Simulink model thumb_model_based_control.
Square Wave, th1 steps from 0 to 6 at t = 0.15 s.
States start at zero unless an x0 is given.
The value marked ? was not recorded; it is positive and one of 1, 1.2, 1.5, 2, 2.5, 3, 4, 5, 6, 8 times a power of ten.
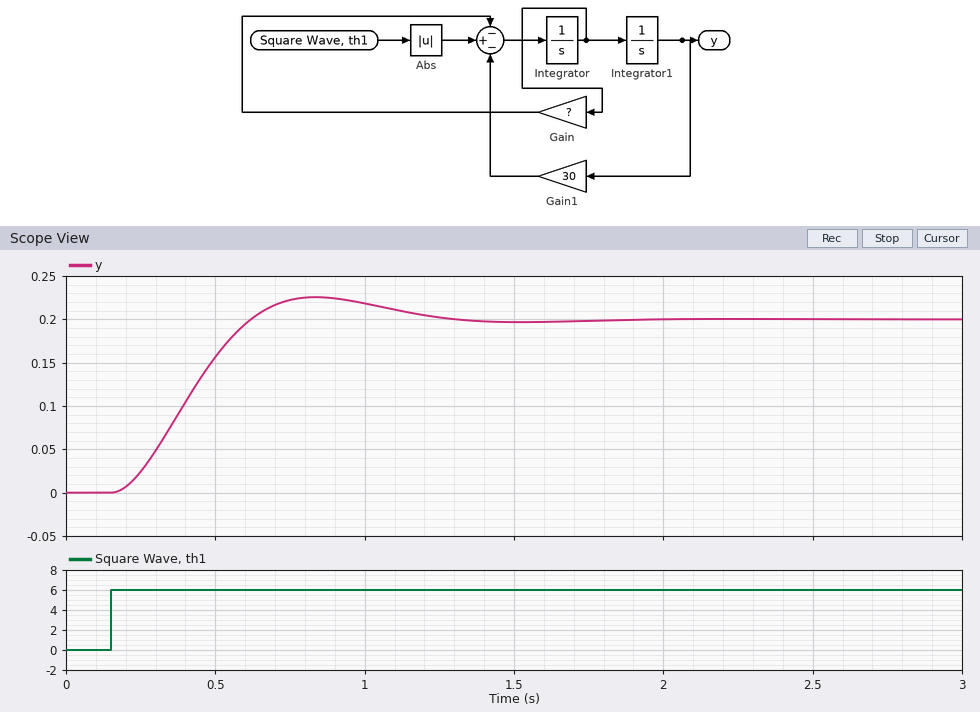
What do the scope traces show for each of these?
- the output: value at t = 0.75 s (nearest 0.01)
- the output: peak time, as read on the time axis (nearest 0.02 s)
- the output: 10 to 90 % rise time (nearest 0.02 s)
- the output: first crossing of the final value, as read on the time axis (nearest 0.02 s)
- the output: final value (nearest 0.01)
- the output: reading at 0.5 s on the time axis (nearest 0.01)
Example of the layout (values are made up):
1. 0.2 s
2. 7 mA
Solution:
1. 0.22
2. 0.84 s
3. 0.32 s
4. 0.62 s
5. 0.20
6. 0.16
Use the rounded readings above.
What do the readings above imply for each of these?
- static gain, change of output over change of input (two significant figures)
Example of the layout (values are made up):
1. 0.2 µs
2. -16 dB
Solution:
1. 0.033
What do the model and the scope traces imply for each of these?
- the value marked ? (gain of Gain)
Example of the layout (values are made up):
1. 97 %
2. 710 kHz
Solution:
1. 6
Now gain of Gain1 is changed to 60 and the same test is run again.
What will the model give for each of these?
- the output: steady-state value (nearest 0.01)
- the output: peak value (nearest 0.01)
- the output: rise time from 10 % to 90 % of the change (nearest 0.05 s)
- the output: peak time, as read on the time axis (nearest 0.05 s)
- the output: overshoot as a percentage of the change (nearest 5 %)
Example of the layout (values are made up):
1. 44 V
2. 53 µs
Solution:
1. 0.10
2. 0.13
3. 0.20 s
4. 0.60 s
5. 25 %
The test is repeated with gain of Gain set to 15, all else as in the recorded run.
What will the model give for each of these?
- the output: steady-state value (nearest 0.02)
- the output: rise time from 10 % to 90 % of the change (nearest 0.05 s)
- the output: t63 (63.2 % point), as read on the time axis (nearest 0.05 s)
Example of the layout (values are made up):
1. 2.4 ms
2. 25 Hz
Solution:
1. 0.20
2. 0.95 s
3. 0.65 s
